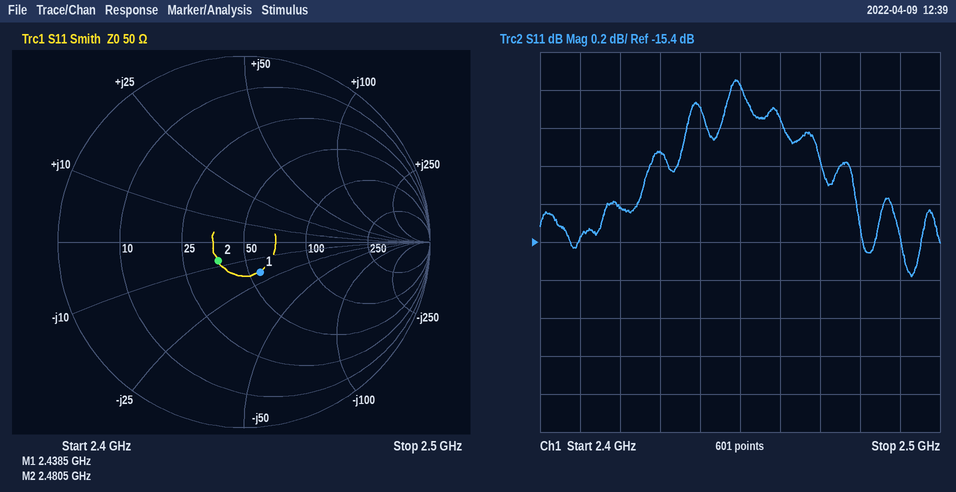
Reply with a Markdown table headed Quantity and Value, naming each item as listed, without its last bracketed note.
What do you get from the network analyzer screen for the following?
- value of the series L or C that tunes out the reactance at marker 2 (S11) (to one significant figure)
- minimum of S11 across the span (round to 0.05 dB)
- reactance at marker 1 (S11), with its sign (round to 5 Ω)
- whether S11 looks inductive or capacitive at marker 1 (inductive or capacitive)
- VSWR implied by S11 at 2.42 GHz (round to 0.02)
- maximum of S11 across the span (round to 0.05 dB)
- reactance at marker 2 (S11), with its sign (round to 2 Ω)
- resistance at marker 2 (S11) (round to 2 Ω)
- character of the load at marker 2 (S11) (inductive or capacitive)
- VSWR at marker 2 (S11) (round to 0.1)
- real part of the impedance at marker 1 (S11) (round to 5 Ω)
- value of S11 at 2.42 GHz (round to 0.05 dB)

| Quantity | Value |
|---|---|
| value of the series L or C that tunes out the reactance at marker 2 (S11) | 500 pH |
| minimum of S11 across the span | -15.60 dB |
| reactance at marker 1 (S11), with its sign | -20 Ω |
| whether S11 looks inductive or capacitive at marker 1 | capacitive |
| VSWR implied by S11 at 2.42 GHz | 1.42 |
| maximum of S11 across the span | -14.55 dB |
| reactance at marker 2 (S11), with its sign | -8 Ω |
| resistance at marker 2 (S11) | 38 Ω |
| character of the load at marker 2 (S11) | capacitive |
| VSWR at marker 2 (S11) | 1.4 |
| real part of the impedance at marker 1 (S11) | 55 Ω |
| value of S11 at 2.42 GHz | -15.20 dB |
